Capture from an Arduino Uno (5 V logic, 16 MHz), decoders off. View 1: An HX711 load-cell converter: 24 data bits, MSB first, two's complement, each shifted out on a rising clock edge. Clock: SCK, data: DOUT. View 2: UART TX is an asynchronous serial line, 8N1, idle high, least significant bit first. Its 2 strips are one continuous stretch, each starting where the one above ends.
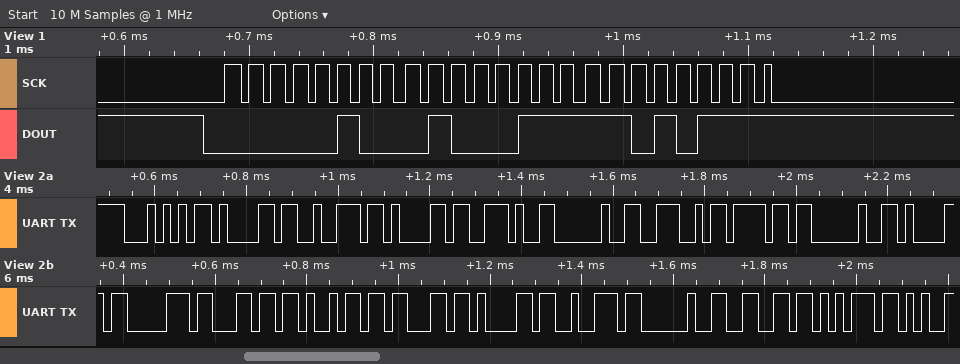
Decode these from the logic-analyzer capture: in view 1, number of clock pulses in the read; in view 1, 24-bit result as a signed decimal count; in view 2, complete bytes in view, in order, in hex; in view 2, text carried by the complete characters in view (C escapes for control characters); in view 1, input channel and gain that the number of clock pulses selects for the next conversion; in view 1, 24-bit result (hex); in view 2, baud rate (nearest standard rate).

25
280535
54 61 72 61 2E 20 4E 6F 20 61 70 6C 69 63 61 72 20 66 75
"Tara. No aplicar fu"
channel A, gain 128
0x0447D7
57600 baud
